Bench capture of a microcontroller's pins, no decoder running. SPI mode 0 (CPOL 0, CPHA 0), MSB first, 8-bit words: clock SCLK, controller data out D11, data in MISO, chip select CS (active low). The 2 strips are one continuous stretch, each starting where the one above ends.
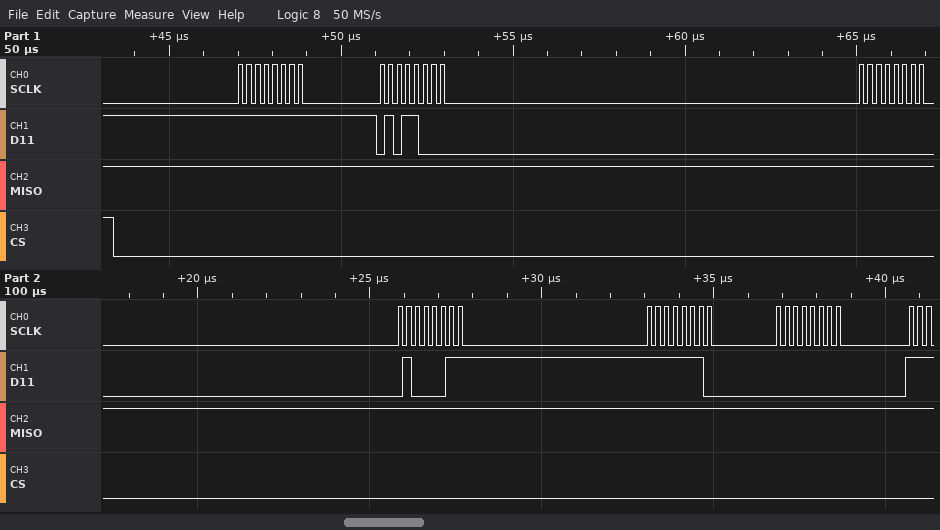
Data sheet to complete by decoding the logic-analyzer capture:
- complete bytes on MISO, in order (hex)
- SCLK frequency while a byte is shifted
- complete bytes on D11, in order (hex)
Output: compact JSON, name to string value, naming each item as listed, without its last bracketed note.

{"complete bytes on MISO, in order": "FF FF FF FF FF FF", "SCLK frequency while a byte is shifted": "4 MHz", "complete bytes on D11, in order": "FF 58 00 43 FE 00"}
